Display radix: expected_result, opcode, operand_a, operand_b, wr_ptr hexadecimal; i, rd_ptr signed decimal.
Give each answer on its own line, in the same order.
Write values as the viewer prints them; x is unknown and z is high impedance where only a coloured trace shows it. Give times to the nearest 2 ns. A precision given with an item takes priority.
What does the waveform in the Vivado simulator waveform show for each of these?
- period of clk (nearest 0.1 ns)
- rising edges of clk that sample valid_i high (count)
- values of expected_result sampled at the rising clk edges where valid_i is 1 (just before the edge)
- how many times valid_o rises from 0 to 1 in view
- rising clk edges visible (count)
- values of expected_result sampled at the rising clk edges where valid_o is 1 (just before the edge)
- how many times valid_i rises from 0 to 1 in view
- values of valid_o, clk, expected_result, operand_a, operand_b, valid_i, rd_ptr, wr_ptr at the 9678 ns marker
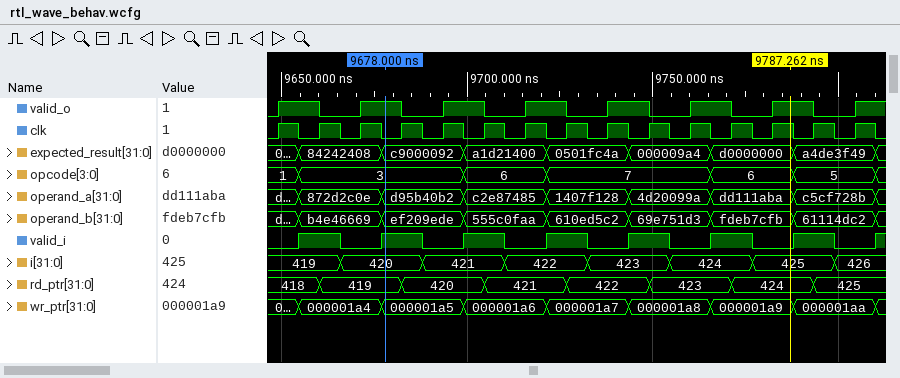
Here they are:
11.1 ns
7
84242408, c9000092, a1d21400, 0501fc4a, 000009a4, d0000000, a4de3f49
8
15
84242408, c9000092, a1d21400, 0501fc4a, 000009a4, d0000000, a4de3f49
8
valid_o=1, clk=0, expected_result=c9000092, operand_a=d95b40b2, operand_b=ef209ede, valid_i=1, rd_ptr=419, wr_ptr=000001a5
